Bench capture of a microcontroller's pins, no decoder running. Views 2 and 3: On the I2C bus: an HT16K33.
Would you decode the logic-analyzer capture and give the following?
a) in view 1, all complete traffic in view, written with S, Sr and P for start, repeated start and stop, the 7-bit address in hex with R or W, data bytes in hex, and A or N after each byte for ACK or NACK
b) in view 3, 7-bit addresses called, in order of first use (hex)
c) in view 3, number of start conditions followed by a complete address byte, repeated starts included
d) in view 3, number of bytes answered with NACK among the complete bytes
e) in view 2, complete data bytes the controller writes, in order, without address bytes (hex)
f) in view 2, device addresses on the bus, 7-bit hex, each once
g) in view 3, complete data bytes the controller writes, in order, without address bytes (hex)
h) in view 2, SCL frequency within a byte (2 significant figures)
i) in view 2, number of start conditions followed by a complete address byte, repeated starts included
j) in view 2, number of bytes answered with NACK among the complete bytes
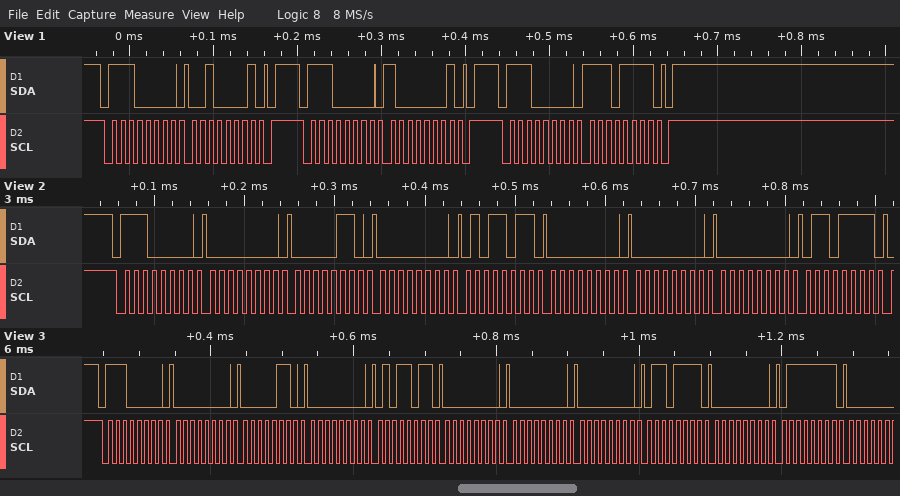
S 70W A 21 A P S 70W A 81 A P S 70W A EF A P
0x70
1
0
00 06 00 5B 00 00 00 6F
0x70
00 06 00 5B 00 00 00 6F 00 7F
100 kHz
1
0
